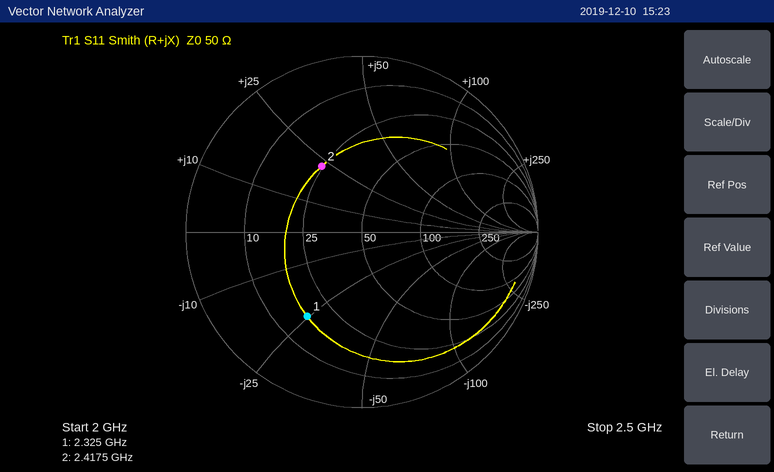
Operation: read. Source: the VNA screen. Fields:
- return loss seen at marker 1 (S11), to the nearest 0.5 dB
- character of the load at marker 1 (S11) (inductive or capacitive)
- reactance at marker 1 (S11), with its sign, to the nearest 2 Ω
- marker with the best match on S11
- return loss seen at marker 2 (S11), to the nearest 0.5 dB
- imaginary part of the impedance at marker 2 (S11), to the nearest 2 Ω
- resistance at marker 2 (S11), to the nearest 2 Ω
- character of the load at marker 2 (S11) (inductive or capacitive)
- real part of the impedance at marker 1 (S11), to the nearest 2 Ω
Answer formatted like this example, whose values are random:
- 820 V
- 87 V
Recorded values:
- 5.0 dB
- capacitive
- -24 Ω
- marker 2
- 7.0 dB
- +22 Ω
- 24 Ω
- inductive
- 18 Ω
